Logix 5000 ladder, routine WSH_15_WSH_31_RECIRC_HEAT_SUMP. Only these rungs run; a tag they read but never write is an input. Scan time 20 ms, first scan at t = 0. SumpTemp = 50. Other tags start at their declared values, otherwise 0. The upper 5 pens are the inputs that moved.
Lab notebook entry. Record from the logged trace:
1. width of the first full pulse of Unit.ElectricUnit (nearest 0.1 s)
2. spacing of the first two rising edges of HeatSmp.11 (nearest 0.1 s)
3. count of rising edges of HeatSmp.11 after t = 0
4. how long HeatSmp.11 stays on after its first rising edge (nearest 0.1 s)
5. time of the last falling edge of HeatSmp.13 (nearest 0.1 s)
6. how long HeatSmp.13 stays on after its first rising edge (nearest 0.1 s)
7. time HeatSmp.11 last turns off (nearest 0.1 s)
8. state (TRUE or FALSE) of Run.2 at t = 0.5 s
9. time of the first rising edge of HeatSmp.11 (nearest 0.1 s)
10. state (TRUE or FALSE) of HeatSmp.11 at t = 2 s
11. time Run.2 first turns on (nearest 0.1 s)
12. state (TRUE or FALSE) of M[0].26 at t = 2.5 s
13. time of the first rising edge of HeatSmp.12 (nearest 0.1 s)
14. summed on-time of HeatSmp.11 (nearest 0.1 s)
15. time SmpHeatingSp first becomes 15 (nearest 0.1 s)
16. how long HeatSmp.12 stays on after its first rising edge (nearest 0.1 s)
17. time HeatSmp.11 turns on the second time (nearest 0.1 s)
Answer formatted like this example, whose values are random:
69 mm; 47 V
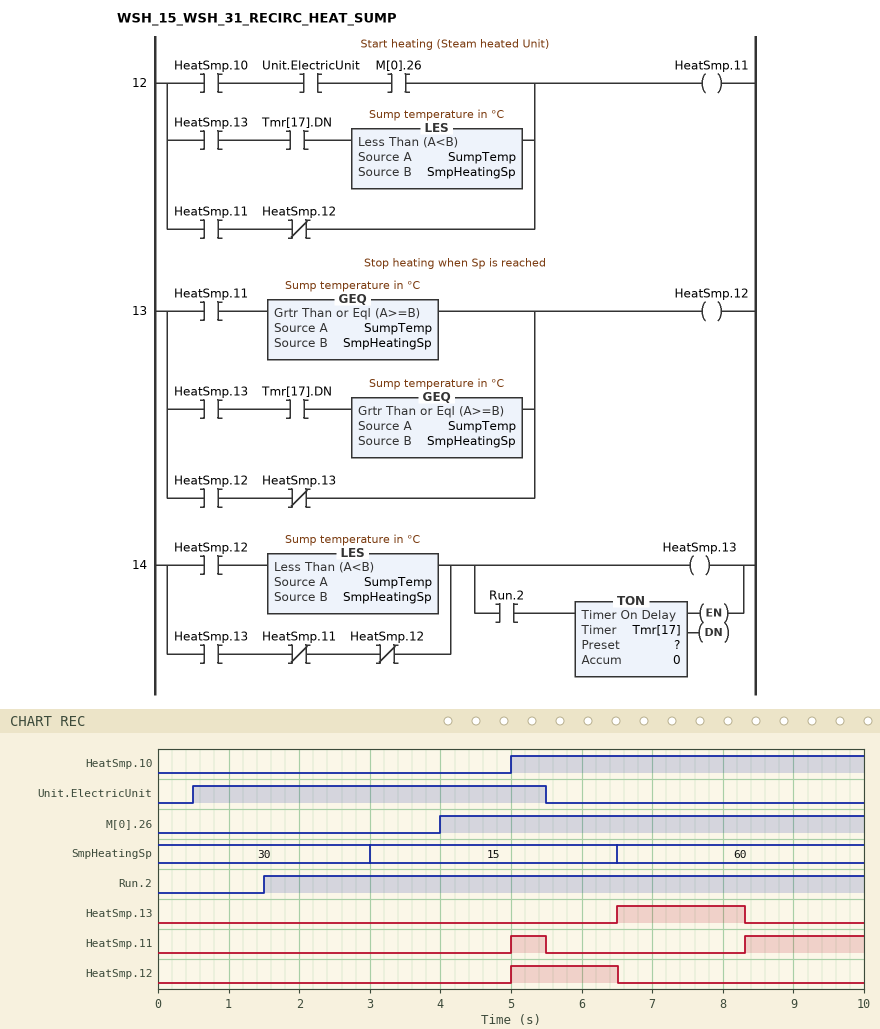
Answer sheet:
5.0 s; 3.3 s; 2; 0.5 s; 8.3 s; 1.8 s; 5.5 s; FALSE; 5.0 s; FALSE; 1.5 s; FALSE; 5.0 s; 2.2 s; 3.0 s; 1.5 s; 8.3 s
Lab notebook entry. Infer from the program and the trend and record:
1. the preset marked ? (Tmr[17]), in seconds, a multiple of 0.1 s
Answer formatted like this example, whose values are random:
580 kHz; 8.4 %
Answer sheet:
1.8 s
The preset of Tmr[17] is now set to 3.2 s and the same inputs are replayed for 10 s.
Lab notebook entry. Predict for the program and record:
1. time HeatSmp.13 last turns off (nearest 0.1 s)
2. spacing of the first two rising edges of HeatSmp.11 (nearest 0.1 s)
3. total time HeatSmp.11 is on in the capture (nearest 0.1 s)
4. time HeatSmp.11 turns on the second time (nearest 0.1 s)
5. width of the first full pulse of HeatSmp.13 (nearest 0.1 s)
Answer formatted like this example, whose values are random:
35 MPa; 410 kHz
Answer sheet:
9.7 s; 4.7 s; 0.8 s; 9.7 s; 3.2 s
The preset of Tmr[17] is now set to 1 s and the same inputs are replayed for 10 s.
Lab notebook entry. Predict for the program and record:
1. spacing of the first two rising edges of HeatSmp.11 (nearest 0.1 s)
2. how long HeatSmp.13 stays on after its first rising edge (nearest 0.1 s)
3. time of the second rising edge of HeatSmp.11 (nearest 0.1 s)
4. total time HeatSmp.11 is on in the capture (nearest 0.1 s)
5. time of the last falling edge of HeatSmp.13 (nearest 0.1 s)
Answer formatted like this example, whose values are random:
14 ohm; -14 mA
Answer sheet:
2.5 s; 1.0 s; 7.5 s; 3.0 s; 7.5 s
